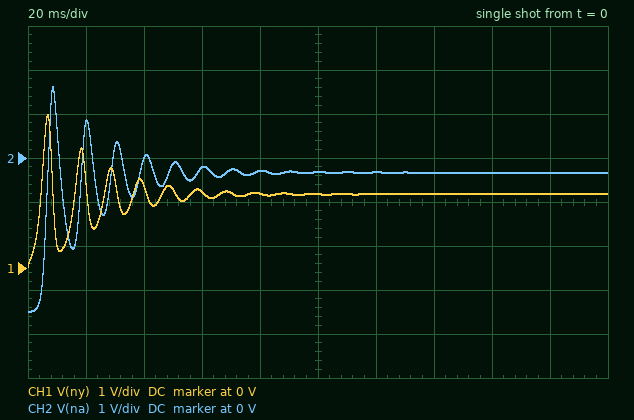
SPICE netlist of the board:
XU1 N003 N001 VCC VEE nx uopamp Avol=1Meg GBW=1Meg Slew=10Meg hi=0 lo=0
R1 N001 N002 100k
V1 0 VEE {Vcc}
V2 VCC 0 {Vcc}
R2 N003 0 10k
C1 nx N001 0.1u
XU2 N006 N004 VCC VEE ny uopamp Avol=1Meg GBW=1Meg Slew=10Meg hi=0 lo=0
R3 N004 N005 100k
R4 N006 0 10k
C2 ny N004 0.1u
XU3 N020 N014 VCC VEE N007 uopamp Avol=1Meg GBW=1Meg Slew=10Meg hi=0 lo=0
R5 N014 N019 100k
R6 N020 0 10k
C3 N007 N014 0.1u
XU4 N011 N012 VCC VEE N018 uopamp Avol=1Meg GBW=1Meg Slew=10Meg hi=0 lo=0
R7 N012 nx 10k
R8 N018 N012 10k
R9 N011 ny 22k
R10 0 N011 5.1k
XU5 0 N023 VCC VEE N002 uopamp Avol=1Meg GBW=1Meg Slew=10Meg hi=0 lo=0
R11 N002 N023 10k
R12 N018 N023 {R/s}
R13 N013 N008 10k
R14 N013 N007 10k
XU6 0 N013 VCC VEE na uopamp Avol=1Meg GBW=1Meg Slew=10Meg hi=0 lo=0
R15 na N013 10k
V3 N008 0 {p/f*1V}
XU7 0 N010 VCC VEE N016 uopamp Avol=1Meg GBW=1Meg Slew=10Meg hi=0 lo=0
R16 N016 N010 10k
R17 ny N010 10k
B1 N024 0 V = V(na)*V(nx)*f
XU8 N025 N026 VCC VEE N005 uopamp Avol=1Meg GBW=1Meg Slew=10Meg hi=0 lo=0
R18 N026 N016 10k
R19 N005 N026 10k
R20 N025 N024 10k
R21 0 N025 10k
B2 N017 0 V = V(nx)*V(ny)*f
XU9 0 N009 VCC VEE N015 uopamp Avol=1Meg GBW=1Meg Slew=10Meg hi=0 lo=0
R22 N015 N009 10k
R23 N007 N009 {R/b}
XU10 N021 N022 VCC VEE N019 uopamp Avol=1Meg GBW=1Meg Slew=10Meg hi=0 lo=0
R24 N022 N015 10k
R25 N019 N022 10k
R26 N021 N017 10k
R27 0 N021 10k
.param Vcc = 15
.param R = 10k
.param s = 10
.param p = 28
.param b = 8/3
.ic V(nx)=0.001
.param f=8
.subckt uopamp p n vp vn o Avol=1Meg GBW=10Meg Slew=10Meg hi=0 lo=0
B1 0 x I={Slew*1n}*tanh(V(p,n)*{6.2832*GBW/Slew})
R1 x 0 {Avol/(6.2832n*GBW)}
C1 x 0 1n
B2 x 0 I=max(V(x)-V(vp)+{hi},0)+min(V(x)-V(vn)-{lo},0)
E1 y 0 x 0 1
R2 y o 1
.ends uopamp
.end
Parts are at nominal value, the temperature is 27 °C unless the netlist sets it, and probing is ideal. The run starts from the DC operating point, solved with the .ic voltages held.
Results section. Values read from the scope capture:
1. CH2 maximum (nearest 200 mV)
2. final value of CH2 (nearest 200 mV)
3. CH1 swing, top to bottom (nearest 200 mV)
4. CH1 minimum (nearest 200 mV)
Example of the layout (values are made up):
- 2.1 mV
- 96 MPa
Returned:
- 1.6 V
- -400 mV
- 3.4 V
- 0 V
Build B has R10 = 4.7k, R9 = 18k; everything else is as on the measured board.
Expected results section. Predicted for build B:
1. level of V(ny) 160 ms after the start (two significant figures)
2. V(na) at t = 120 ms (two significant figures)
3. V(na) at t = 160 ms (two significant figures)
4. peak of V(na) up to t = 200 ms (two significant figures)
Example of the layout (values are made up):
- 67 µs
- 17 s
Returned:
- 1.6 V
- -310 mV
- -300 mV
- 1.8 V
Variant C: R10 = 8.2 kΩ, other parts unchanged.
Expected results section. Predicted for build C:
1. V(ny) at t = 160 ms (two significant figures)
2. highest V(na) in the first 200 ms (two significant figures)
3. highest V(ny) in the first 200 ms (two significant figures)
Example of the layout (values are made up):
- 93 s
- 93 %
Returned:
- -1.4 V
- 2.3 V
- 3.9 V
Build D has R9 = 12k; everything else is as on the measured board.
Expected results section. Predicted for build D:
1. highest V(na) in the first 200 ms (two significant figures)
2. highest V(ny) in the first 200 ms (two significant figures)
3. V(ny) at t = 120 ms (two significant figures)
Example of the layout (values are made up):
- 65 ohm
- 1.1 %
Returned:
- 2.5 V
- 4.0 V
- -1.4 V
